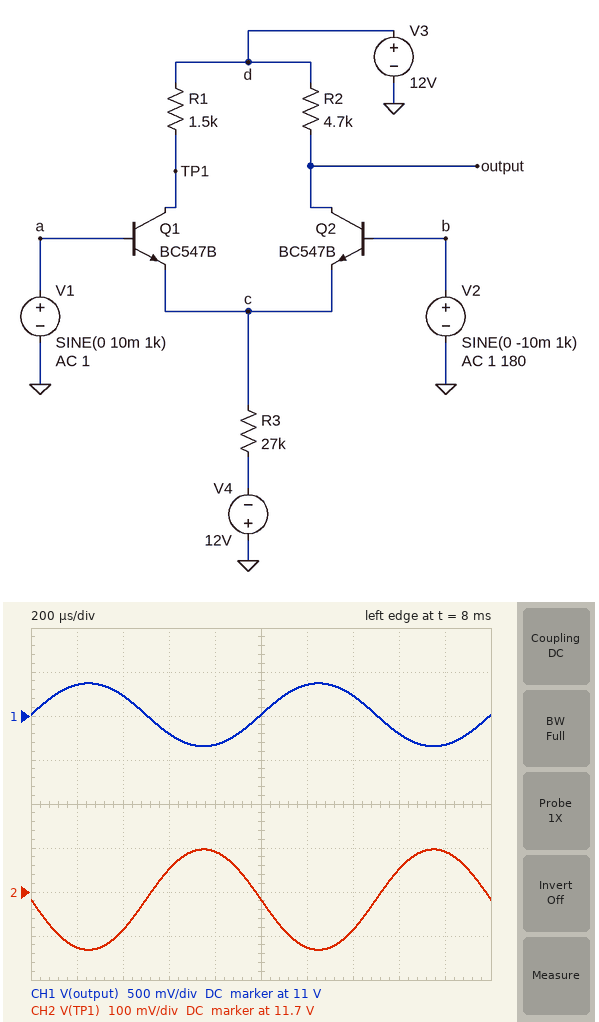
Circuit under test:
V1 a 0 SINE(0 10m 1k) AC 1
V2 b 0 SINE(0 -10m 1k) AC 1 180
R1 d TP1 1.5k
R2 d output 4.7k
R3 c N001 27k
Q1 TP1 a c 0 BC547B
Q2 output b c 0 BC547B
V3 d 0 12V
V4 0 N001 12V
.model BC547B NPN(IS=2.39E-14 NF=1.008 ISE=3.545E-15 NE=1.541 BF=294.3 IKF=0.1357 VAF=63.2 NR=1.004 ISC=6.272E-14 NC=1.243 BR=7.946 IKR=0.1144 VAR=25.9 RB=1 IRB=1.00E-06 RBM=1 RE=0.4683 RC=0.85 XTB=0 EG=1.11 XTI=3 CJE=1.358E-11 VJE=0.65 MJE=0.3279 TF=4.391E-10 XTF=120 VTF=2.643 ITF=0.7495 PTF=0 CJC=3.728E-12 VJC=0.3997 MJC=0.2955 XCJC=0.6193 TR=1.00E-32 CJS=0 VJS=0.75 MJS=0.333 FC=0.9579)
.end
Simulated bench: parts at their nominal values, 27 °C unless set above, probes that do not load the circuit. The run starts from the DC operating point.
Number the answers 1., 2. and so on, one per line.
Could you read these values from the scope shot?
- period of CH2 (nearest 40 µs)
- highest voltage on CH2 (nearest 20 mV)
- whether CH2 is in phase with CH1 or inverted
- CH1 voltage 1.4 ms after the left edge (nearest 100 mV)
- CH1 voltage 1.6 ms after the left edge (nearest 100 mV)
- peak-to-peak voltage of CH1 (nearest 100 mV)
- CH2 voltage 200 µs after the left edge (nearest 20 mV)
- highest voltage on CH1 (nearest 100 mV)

1. 1.00 ms
2. 11.80 V
3. inverted
4. 11.2 V
5. 10.8 V
6. 700 mV
7. 11.58 V
8. 11.4 V
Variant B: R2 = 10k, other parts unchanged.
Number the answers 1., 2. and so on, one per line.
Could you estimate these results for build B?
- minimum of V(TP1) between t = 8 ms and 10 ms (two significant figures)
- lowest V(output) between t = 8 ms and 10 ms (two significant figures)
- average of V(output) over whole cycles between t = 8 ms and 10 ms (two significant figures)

1. 12 V
2. 9.2 V
3. 9.9 V
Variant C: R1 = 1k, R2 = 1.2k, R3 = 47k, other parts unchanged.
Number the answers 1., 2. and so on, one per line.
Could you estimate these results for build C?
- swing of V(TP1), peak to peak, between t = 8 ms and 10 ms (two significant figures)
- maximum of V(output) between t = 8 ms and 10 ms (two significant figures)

1. 88 mV
2. 12 V
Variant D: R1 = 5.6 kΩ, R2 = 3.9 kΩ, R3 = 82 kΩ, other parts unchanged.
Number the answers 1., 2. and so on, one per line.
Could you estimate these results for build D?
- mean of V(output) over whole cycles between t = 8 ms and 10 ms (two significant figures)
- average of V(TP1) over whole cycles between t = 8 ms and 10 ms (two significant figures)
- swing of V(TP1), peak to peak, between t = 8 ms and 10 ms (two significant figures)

1. 12 V
2. 12 V
3. 280 mV
